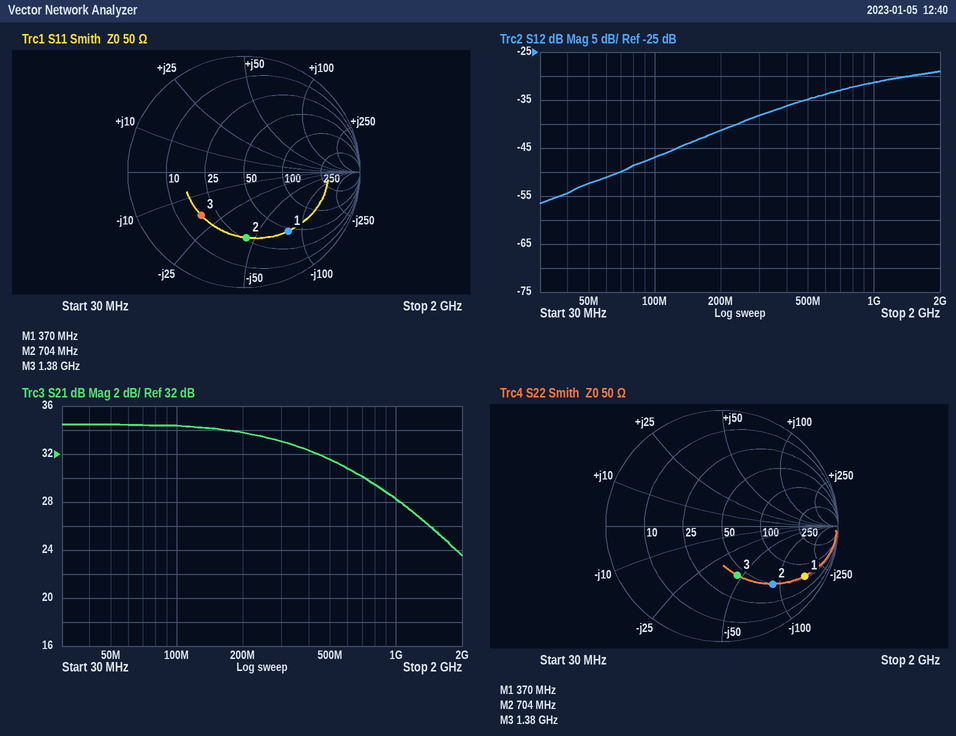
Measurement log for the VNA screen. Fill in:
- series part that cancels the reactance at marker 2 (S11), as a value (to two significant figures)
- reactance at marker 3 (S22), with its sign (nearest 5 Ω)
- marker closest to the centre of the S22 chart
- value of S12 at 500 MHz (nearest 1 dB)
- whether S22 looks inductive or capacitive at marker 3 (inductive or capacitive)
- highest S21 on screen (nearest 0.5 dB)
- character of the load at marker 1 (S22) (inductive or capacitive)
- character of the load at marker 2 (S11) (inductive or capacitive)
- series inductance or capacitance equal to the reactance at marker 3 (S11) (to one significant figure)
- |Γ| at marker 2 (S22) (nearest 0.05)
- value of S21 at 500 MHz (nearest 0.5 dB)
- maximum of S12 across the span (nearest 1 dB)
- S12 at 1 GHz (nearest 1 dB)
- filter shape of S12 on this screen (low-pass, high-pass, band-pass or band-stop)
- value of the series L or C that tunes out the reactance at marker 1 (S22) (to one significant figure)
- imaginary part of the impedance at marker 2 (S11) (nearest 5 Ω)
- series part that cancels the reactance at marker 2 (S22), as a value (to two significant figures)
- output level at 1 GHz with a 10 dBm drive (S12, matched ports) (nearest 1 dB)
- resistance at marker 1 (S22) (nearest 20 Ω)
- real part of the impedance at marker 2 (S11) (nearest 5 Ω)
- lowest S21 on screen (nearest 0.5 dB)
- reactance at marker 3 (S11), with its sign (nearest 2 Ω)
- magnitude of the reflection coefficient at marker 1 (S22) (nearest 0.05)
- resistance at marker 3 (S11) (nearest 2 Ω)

10 nH
-45 Ω
marker 3
-35 dB
capacitive
34.5 dB
capacitive
capacitive
6 pF
0.65
31.5 dB
-29 dB
-31 dB
high-pass
70 nH
-45 Ω
20 nH
-21 dBm
60 Ω
25 Ω
23.5 dB
-18 Ω
0.85
18 Ω
